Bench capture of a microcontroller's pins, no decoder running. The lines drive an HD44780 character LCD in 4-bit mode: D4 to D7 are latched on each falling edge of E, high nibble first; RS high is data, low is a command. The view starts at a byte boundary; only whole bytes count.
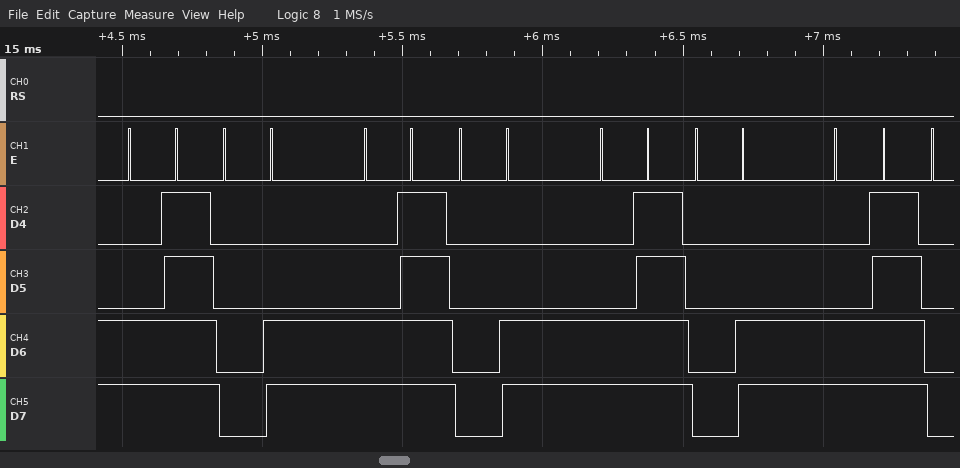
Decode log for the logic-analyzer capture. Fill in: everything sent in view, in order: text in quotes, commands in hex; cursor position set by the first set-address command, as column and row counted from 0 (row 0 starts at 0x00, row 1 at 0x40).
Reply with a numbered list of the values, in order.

1. 0xCF 0x0C 0xCF 0x0C 0xCF 0x0C 0xCF
2. column 15, row 1
